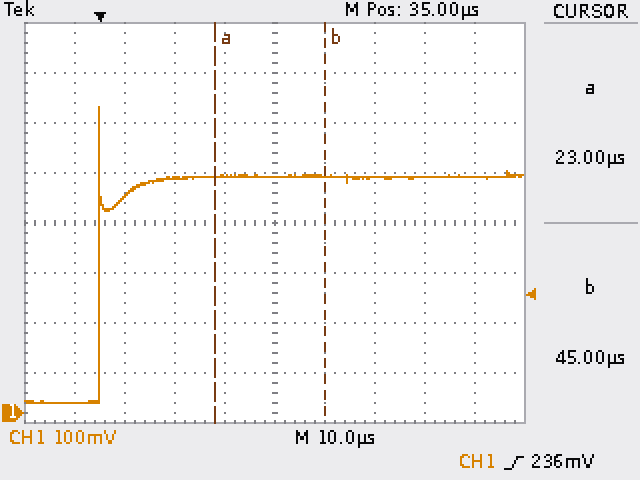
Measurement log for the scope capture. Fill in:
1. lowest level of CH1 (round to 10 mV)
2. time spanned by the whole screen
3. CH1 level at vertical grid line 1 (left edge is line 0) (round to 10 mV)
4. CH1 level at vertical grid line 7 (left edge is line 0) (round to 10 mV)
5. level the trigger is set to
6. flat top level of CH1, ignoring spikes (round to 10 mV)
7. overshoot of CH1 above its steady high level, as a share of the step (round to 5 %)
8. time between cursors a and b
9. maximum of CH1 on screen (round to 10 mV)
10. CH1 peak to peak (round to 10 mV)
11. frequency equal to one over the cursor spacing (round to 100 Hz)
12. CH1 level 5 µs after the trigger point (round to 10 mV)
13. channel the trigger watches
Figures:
20 mV
100 µs
20 mV
470 mV
236 mV
470 mV
30 %
22 µs
610 mV
590 mV
45.5 kHz
430 mV
CH1
